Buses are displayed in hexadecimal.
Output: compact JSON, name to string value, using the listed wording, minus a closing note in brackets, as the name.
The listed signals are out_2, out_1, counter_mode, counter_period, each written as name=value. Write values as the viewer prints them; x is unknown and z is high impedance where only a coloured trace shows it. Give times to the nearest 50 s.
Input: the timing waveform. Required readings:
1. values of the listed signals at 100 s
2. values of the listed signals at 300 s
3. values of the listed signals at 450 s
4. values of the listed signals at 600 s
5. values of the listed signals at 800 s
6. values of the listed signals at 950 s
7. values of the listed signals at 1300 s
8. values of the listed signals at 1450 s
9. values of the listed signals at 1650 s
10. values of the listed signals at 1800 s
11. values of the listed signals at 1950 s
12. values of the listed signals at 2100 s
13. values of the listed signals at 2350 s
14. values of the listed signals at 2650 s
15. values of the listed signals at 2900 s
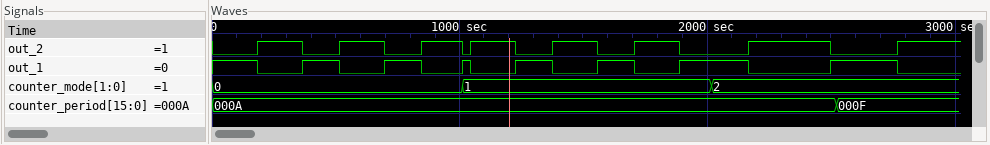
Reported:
{"values of the listed signals at 100 s": "out_2=0, out_1=1, counter_mode=0, counter_period=000A", "values of the listed signals at 300 s": "out_2=1, out_1=0, counter_mode=0, counter_period=000A", "values of the listed signals at 450 s": "out_2=0, out_1=1, counter_mode=0, counter_period=000A", "values of the listed signals at 600 s": "out_2=1, out_1=0, counter_mode=0, counter_period=000A", "values of the listed signals at 800 s": "out_2=0, out_1=1, counter_mode=0, counter_period=000A", "values of the listed signals at 950 s": "out_2=1, out_1=0, counter_mode=0, counter_period=000A", "values of the listed signals at 1300 s": "out_2=0, out_1=1, counter_mode=1, counter_period=000A", "values of the listed signals at 1450 s": "out_2=1, out_1=0, counter_mode=1, counter_period=000A", "values of the listed signals at 1650 s": "out_2=0, out_1=1, counter_mode=1, counter_period=000A", "values of the listed signals at 1800 s": "out_2=1, out_1=0, counter_mode=1, counter_period=000A", "values of the listed signals at 1950 s": "out_2=0, out_1=1, counter_mode=1, counter_period=000A", "values of the listed signals at 2100 s": "out_2=0, out_1=1, counter_mode=2, counter_period=000A", "values of the listed signals at 2350 s": "out_2=1, out_1=0, counter_mode=2, counter_period=000A", "values of the listed signals at 2650 s": "out_2=0, out_1=1, counter_mode=2, counter_period=000F", "values of the listed signals at 2900 s": "out_2=1, out_1=0, counter_mode=2, counter_period=000F"}
